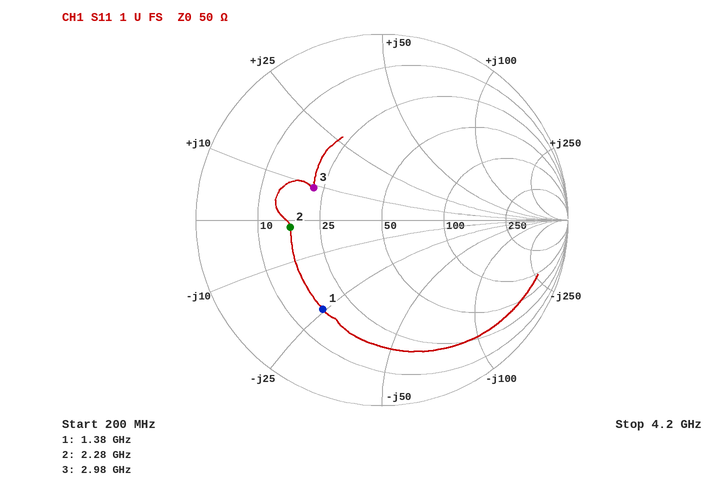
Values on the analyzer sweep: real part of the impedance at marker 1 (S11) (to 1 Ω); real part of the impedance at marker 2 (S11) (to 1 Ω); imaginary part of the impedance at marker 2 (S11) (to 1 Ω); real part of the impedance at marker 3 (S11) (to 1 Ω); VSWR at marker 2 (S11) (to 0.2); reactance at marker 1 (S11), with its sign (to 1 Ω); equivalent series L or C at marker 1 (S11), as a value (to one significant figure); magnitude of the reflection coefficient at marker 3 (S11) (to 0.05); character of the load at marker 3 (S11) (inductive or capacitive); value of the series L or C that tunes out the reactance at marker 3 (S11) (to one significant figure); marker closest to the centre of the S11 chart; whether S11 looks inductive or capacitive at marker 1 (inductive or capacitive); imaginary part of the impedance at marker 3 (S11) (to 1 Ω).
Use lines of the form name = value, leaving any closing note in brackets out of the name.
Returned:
real part of the impedance at marker 1 (S11) = 17 Ω
real part of the impedance at marker 2 (S11) = 17 Ω
imaginary part of the impedance at marker 2 (S11) = -2 Ω
real part of the impedance at marker 3 (S11) = 22 Ω
VSWR at marker 2 (S11) = 3.0
reactance at marker 1 (S11), with its sign = -24 Ω
equivalent series L or C at marker 1 (S11), as a value = 5 pF
magnitude of the reflection coefficient at marker 3 (S11) = 0.40
character of the load at marker 3 (S11) = inductive
value of the series L or C that tunes out the reactance at marker 3 (S11) = 6 pF
marker closest to the centre of the S11 chart = marker 3
whether S11 looks inductive or capacitive at marker 1 = capacitive
imaginary part of the impedance at marker 3 (S11) = +9 Ω
